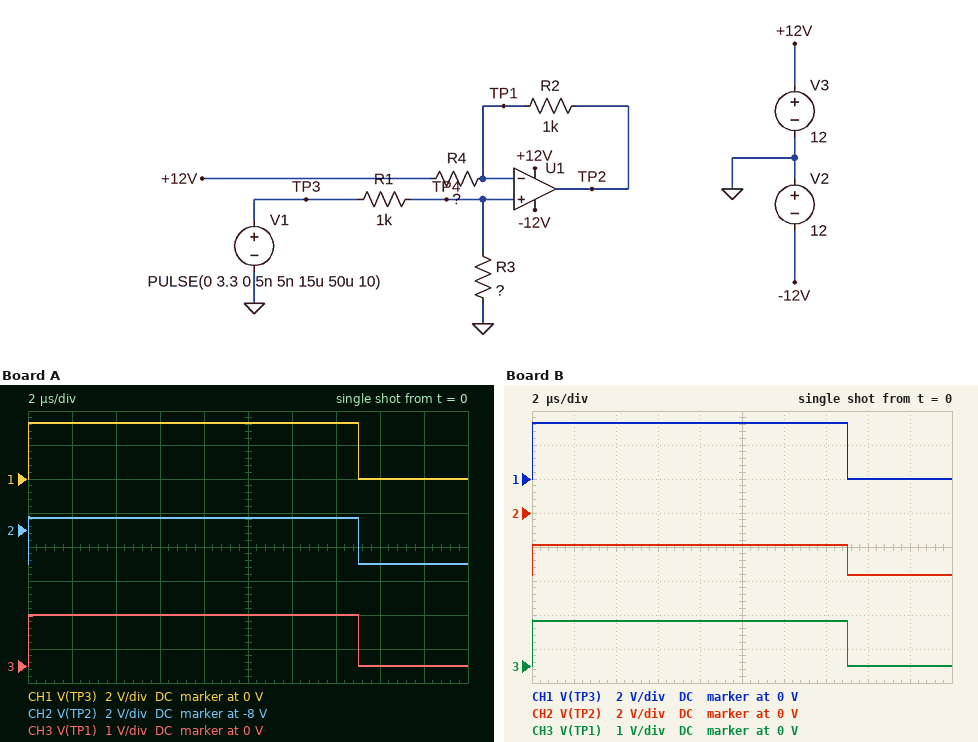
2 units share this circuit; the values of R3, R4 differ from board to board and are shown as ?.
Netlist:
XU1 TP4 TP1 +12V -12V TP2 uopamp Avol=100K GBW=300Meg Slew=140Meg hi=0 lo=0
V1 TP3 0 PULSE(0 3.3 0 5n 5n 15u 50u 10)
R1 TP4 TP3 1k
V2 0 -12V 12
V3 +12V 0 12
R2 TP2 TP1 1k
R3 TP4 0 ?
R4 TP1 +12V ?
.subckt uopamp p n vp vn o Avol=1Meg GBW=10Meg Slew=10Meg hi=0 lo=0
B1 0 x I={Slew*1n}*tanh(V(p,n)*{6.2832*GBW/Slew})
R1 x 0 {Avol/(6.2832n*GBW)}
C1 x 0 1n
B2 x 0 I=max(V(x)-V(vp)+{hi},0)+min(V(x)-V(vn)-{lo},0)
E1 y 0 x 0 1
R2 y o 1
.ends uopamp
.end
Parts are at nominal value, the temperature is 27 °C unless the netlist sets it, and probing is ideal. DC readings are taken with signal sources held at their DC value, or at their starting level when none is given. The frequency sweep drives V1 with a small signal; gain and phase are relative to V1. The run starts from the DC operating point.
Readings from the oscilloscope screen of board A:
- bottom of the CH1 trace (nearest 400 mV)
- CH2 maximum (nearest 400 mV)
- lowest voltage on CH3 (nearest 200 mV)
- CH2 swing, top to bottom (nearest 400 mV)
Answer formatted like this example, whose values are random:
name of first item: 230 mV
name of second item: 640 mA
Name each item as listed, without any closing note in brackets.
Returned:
bottom of the CH1 trace: 0 V
CH2 maximum: -7.2 V
lowest voltage on CH3: 0 V
CH2 swing, top to bottom: 2.8 V
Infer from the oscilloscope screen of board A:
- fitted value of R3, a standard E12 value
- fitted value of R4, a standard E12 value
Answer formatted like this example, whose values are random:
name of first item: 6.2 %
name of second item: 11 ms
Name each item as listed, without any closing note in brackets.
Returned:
fitted value of R3, a standard E12 value: 820 Ω
fitted value of R4, a standard E12 value: 1.2 kΩ
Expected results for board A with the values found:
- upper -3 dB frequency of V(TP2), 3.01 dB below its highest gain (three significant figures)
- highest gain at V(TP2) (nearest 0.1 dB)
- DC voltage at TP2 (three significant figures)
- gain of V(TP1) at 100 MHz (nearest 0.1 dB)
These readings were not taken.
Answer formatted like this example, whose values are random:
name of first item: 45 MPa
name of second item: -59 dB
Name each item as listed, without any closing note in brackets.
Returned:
upper -3 dB frequency of V(TP2), 3.01 dB below its highest gain: 164 MHz
highest gain at V(TP2): -1.7 dB
DC voltage at TP2: -10.0 V
gain of V(TP1) at 100 MHz: -8.3 dB
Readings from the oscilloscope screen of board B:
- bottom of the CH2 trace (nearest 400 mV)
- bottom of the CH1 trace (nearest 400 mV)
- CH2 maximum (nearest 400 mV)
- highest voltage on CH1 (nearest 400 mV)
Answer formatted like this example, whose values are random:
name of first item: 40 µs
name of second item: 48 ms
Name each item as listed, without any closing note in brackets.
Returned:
bottom of the CH2 trace: -3.6 V
bottom of the CH1 trace: 0 V
CH2 maximum: -2.0 V
highest voltage on CH1: 3.2 V
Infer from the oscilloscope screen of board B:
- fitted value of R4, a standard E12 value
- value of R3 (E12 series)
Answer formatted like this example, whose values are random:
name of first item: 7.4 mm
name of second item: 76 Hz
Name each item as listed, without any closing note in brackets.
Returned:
fitted value of R4, a standard E12 value: 3.3 kΩ
value of R3: 680 Ω
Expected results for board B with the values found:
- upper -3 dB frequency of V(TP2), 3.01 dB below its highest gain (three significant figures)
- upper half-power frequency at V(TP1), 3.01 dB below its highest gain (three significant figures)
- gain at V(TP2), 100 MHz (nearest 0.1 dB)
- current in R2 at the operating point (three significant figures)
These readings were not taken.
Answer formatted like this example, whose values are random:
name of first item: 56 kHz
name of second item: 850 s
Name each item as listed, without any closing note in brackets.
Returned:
upper -3 dB frequency of V(TP2), 3.01 dB below its highest gain: 230 MHz
upper half-power frequency at V(TP1), 3.01 dB below its highest gain: 230 MHz
gain at V(TP2), 100 MHz: -6.3 dB
current in R2 at the operating point: 3.64 mA
